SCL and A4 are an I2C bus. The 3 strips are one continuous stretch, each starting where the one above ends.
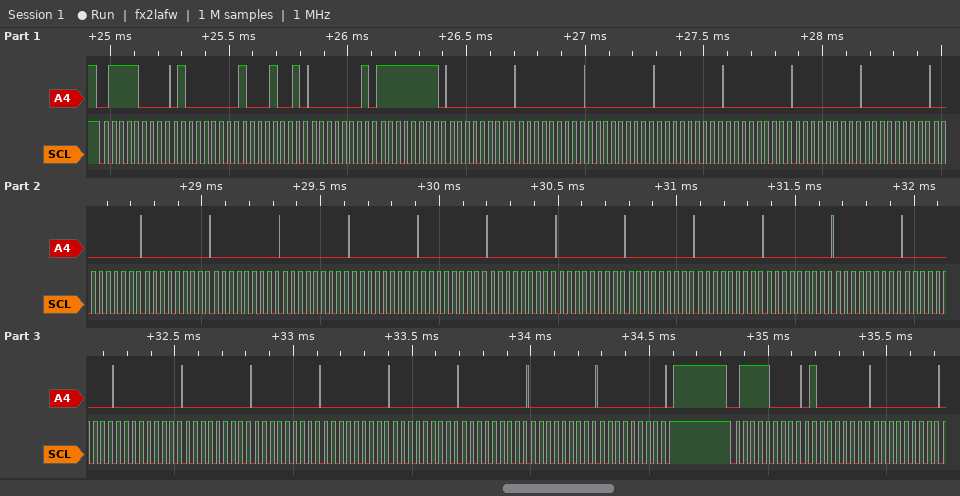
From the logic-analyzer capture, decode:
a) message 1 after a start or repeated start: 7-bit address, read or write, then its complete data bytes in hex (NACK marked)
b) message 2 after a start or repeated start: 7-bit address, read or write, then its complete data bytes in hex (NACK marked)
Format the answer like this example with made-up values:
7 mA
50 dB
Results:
0x3C write: 40 89 01 FF 00 00 00 00 00 00 00 00 00 00 00 00 00 00 00 00 00 00 00 00 00 00 00 00 00 00 00 00
0x3C write: 40 00
